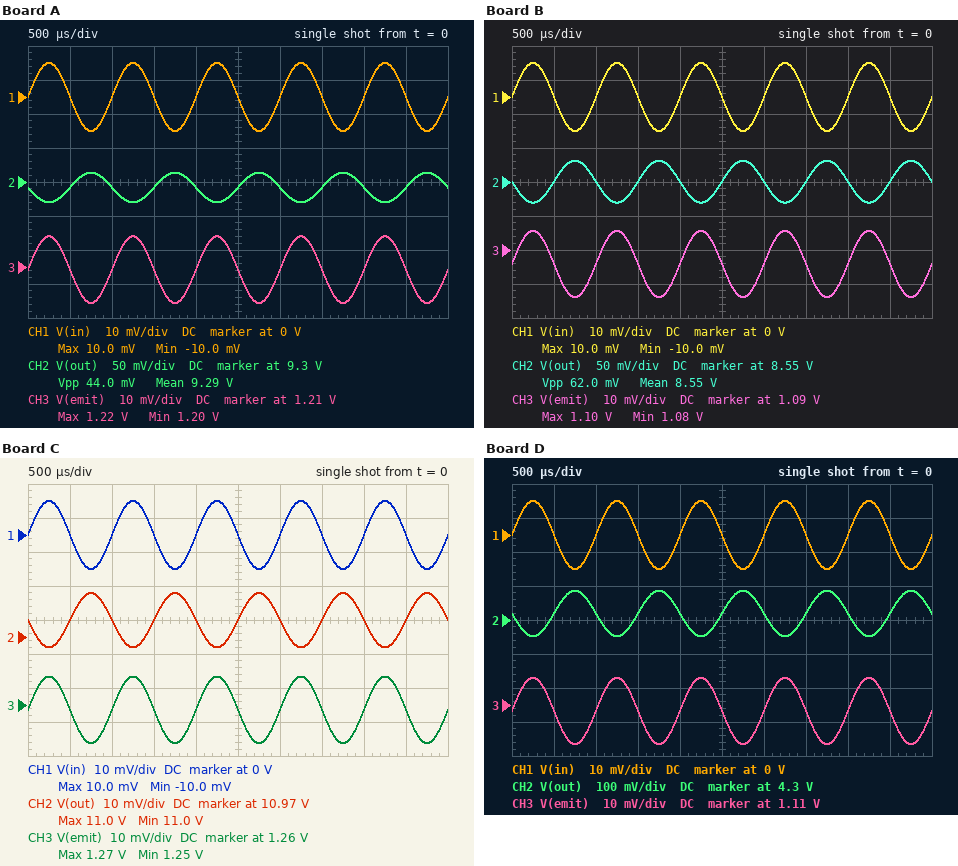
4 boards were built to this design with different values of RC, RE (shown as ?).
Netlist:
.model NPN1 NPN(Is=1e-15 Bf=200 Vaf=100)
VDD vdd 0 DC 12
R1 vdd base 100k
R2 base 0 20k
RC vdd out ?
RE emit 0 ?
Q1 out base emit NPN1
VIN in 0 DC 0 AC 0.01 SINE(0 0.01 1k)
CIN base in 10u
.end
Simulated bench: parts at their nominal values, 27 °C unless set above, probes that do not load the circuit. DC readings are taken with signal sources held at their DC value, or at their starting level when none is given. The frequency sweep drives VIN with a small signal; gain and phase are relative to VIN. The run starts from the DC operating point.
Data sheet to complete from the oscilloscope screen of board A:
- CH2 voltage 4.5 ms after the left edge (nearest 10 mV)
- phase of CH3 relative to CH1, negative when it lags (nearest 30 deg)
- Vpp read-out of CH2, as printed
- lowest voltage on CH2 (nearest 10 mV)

9.29 V
0 deg
44.0 mV
9.27 V
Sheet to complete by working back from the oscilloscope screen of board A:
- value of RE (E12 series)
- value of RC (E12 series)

1.2 kΩ
2.7 kΩ
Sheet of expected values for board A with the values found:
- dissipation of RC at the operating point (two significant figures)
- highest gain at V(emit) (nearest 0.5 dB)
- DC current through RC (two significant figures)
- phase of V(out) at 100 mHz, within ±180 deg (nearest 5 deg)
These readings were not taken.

2.7 mW
0 dB
1.0 mA
-95 deg
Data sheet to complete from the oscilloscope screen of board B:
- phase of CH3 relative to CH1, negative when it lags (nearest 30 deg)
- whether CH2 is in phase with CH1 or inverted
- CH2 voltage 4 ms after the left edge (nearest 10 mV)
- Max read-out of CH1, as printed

0 deg
inverted
8.55 V
10.0 mV
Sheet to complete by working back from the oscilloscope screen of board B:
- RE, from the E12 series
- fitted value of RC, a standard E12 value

470 Ω
1.5 kΩ
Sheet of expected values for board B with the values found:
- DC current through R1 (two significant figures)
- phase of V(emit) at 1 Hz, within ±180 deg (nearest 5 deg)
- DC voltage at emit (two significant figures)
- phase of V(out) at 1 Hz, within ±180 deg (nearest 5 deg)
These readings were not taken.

100 µA
50 deg
1.1 V
-130 deg
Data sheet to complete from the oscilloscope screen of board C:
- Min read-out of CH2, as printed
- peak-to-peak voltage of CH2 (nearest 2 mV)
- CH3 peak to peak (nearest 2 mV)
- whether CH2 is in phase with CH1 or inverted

11.0 V
16 mV
20 mV
inverted
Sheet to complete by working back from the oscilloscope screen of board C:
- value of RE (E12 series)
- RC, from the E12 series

2.2 kΩ
1.8 kΩ
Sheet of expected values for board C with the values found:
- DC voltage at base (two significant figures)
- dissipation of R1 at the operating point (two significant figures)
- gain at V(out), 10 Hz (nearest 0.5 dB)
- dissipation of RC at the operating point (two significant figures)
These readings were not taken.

2.0 V
1.0 mW
-2.0 dB
580 µW
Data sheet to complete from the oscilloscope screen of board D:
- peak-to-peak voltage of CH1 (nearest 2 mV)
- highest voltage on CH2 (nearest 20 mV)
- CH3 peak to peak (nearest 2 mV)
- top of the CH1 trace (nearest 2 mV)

20 mV
4.38 V
20 mV
10 mV
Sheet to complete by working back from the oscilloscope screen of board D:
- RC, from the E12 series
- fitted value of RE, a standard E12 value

3.9 kΩ
560 Ω
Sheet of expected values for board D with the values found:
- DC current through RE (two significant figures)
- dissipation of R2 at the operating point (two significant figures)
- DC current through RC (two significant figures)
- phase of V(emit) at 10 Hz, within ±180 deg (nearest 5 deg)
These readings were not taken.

2.0 mA
170 µW
2.0 mA
5 deg
